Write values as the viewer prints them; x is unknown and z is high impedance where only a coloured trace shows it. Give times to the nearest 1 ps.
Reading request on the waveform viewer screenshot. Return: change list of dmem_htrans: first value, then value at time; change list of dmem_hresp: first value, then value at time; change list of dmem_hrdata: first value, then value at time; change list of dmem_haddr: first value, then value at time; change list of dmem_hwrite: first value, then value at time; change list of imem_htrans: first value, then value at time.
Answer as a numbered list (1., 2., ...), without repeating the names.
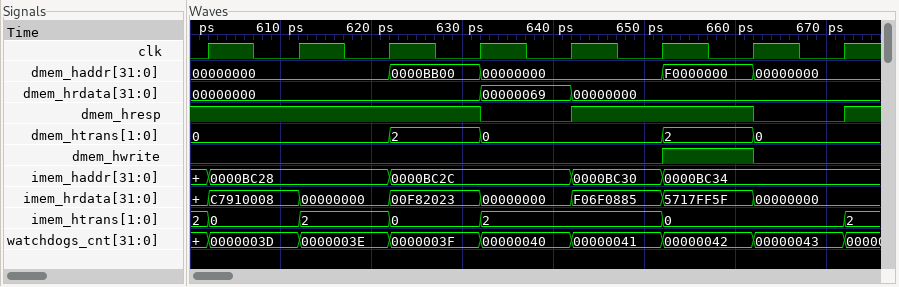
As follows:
1. 0, 2 at 622 ps, 0 at 632 ps, 2 at 652 ps, 0 at 662 ps
2. 1, 0 at 632 ps, 1 at 642 ps, 0 at 662 ps, 1 at 672 ps
3. 00000000, 00000069 at 632 ps, 00000000 at 642 ps
4. 00000000, 0000BB00 at 622 ps, 00000000 at 632 ps, F0000000 at 652 ps, 00000000 at 662 ps
5. 0, 1 at 652 ps, 0 at 662 ps
6. 2, 0 at 602 ps, 2 at 612 ps, 0 at 622 ps, 2 at 632 ps, 0 at 652 ps, 2 at 672 ps
